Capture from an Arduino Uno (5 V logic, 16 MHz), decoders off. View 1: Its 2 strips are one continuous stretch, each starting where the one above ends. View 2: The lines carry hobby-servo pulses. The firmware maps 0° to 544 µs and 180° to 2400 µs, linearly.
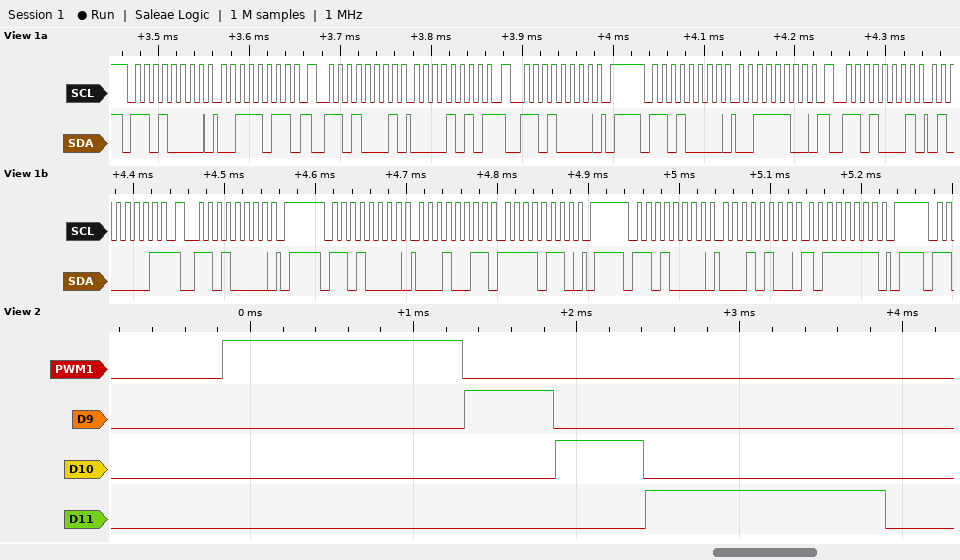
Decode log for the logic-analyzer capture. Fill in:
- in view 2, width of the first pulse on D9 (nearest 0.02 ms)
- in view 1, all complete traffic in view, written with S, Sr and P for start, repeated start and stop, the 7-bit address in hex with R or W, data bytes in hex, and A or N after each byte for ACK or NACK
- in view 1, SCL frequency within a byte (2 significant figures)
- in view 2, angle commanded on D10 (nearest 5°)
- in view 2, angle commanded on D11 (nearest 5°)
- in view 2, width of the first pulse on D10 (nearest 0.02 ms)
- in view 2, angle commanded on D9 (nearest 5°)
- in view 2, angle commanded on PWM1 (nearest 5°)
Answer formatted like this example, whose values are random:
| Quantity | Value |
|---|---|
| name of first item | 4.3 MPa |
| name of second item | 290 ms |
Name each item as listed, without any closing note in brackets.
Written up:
| Quantity | Value |
|---|---|
| in view 2, width of the first pulse on D9 | 0.54 ms |
| in view 1, all complete traffic in view, written with S, Sr and P for start, repeated start and stop, the 7-bit address in hex with R or W, data bytes in hex, and A or N after each byte for ACK or NACK | S 68W A 3B A Sr 68R A 0A N Sr 68W A P S 68W A 3C A Sr 68R A 41 N Sr 68W A P S 68W A 13 A F6 A P S 68W A 14 A BF A P |
| in view 1, SCL frequency within a byte | 100 kHz |
| in view 2, angle commanded on D10 | 0° |
| in view 2, angle commanded on D11 | 90° |
| in view 2, width of the first pulse on D10 | 0.54 ms |
| in view 2, angle commanded on D9 | 0° |
| in view 2, angle commanded on PWM1 | 90° |
